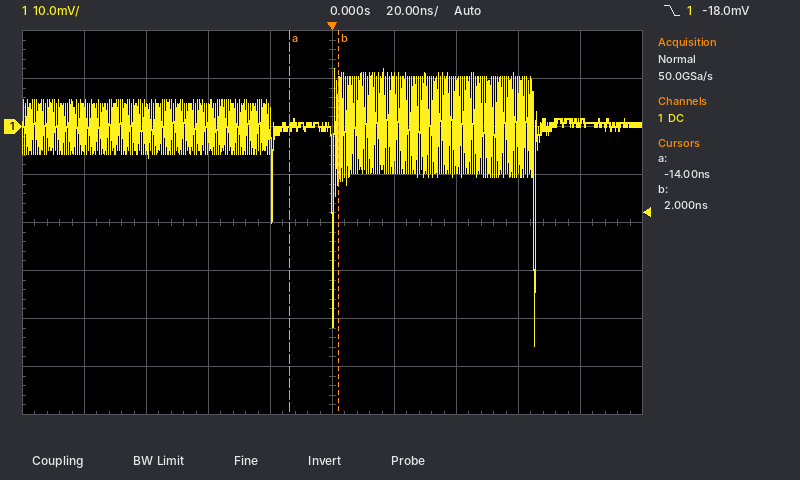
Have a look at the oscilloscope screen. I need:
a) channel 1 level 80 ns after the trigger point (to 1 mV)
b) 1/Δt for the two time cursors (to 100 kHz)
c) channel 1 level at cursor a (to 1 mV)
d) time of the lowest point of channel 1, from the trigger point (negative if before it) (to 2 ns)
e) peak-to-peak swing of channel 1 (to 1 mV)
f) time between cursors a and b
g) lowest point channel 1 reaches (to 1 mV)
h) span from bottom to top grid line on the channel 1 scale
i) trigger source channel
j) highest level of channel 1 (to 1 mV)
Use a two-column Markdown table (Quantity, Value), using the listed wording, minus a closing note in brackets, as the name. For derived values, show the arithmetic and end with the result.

| Quantity | Value |
|---|---|
| channel 1 level 80 ns after the trigger point | 1 mV |
| 1/Δt for the two time cursors | 1 / 16 ns ≈ 62.5 MHz |
| channel 1 level at cursor a | 0 mV |
| time of the lowest point of channel 1, from the trigger point (negative if before it) | +66 ns |
| peak-to-peak swing of channel 1 | 12 mV − (-46 mV) = 58 mV |
| time between cursors a and b | 2 ns − (-14 ns) = 16 ns |
| lowest point channel 1 reaches | -46 mV |
| span from bottom to top grid line on the channel 1 scale | 80 mV |
| trigger source channel | channel 1 |
| highest level of channel 1 | 12 mV |
